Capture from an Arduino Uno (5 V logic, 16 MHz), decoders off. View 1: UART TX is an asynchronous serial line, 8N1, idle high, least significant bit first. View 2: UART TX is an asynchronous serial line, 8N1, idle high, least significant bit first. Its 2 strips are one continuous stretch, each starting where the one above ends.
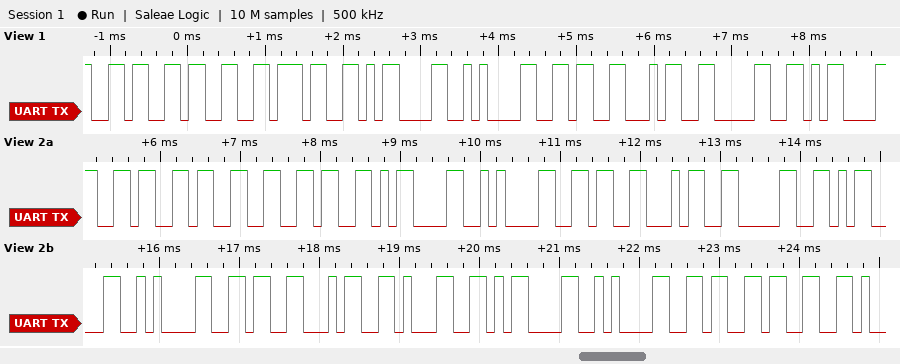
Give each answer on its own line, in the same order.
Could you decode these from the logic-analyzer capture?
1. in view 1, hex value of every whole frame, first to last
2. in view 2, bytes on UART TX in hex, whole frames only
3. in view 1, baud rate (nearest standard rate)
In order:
36 33 37 0D 0A 36 34 30 0D
36 33 36 0D 0A 36 34 30 0D 0A 36 34 31 0D 0A 36 33
9600 baud
